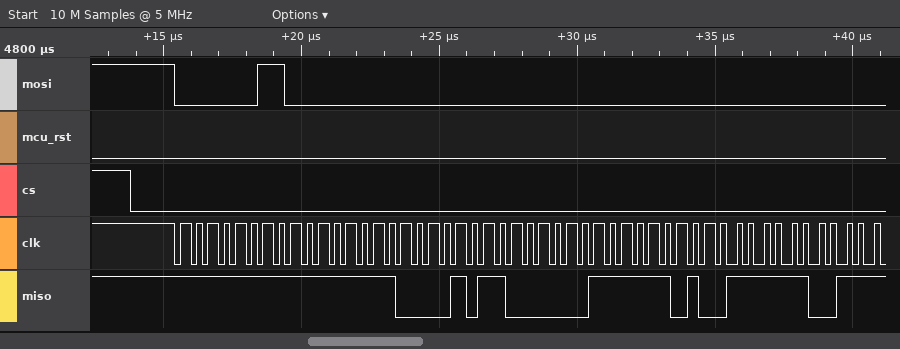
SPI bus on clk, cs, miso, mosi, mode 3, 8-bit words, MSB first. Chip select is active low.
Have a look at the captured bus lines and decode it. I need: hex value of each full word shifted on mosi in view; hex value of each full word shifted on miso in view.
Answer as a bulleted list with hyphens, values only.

- 03, 00, 00, 00, 00, 00
- FF, FF, 0B, 03, F4, FC
